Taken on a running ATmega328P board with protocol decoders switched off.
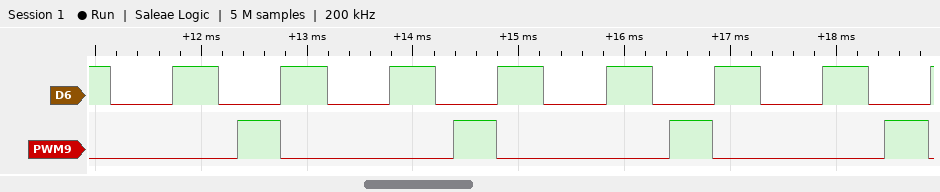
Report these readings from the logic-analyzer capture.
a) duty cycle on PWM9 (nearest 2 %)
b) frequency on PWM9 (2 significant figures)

20 %
490 Hz
